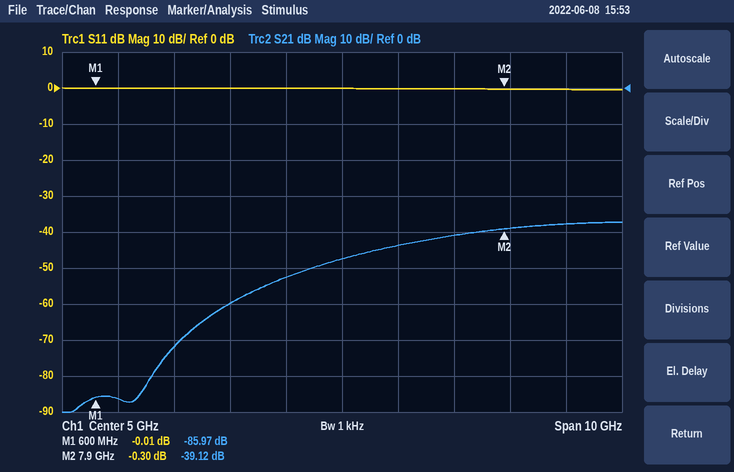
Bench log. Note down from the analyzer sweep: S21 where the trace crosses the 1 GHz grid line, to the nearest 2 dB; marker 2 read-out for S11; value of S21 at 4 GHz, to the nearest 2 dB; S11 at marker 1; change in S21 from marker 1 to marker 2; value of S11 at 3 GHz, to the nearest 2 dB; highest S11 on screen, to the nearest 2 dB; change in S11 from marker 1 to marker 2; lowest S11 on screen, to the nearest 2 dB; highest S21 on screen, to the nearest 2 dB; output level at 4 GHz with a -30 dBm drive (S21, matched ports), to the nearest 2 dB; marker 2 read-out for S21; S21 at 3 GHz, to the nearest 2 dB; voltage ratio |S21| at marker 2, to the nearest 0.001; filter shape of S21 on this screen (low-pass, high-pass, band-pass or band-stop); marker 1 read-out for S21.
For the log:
-86 dB
-0.30 dB
-52 dB
-0.01 dB
46.85 dB
0 dB
0 dB
-0.29 dB
0 dB
-38 dB
-82 dBm
-39.12 dB
-60 dB
0.011
high-pass
-85.97 dB
